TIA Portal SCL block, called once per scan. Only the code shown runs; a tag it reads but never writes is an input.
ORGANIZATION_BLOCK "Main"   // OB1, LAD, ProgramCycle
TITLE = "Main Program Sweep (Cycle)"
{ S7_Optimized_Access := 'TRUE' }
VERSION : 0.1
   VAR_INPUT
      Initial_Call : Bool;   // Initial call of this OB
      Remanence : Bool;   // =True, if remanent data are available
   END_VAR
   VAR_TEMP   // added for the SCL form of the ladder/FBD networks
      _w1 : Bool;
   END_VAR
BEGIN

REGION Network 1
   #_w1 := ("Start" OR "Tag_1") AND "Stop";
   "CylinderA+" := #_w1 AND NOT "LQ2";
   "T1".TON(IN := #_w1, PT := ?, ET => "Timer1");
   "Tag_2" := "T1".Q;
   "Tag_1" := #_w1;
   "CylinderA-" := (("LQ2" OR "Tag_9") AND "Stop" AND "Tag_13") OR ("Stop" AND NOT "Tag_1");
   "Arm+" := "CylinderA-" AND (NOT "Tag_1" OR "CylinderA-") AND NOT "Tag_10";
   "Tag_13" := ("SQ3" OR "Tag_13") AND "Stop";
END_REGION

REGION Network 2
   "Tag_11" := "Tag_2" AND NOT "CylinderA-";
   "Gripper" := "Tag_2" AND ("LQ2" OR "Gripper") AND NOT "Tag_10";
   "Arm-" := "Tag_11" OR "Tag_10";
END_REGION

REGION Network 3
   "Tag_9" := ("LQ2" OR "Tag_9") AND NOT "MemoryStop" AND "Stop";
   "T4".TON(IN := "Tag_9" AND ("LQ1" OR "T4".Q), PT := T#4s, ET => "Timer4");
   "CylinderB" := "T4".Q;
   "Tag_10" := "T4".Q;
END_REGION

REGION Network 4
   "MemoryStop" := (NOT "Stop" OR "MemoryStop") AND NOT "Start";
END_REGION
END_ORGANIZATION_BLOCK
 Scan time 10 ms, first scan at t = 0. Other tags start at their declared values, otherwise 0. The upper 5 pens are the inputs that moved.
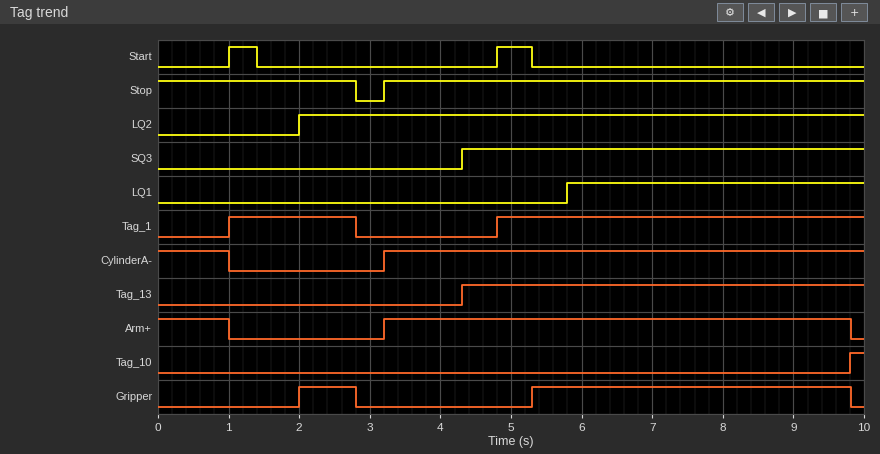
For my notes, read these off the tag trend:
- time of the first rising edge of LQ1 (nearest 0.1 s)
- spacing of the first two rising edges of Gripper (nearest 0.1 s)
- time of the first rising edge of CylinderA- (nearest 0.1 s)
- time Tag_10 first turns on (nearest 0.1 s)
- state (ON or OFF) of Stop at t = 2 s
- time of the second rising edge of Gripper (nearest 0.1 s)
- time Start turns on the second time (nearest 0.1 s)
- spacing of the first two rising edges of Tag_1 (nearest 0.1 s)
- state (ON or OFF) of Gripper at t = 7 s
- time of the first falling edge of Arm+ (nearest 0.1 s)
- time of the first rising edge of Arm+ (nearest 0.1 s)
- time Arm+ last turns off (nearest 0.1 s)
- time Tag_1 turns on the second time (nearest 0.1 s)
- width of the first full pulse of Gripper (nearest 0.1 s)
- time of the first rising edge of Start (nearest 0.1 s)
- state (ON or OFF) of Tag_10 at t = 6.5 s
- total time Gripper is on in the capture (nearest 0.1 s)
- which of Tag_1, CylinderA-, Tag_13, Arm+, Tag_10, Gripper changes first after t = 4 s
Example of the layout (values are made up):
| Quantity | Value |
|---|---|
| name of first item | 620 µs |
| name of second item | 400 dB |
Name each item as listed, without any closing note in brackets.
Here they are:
| Quantity | Value |
|---|---|
| time of the first rising edge of LQ1 | 5.8 s |
| spacing of the first two rising edges of Gripper | 3.3 s |
| time of the first rising edge of CylinderA- | 3.2 s |
| time Tag_10 first turns on | 9.8 s |
| state (ON or OFF) of Stop at t = 2 s | ON |
| time of the second rising edge of Gripper | 5.3 s |
| time Start turns on the second time | 4.8 s |
| spacing of the first two rising edges of Tag_1 | 3.8 s |
| state (ON or OFF) of Gripper at t = 7 s | ON |
| time of the first falling edge of Arm+ | 1.0 s |
| time of the first rising edge of Arm+ | 3.2 s |
| time Arm+ last turns off | 9.8 s |
| time Tag_1 turns on the second time | 4.8 s |
| width of the first full pulse of Gripper | 0.8 s |
| time of the first rising edge of Start | 1.0 s |
| state (ON or OFF) of Tag_10 at t = 6.5 s | OFF |
| total time Gripper is on in the capture | 5.3 s |
| which of Tag_1, CylinderA-, Tag_13, Arm+, Tag_10, Gripper changes first after t = 4 s | Tag_13 |
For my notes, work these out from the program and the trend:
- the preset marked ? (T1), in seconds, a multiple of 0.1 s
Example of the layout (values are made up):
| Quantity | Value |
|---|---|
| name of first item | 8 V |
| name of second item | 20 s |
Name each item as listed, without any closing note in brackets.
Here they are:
| Quantity | Value |
|---|---|
| the preset marked ? (T1), in seconds, a multiple of 0.1 s | 0.5 s |
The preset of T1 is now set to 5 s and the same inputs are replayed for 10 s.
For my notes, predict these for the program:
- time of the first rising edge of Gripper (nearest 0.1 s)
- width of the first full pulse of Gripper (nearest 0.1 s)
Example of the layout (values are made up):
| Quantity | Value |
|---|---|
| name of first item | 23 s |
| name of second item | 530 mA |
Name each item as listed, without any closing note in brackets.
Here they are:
| Quantity | Value |
|---|---|
| time of the first rising edge of Gripper | 9.8 s |
| width of the first full pulse of Gripper | 0.0 s |
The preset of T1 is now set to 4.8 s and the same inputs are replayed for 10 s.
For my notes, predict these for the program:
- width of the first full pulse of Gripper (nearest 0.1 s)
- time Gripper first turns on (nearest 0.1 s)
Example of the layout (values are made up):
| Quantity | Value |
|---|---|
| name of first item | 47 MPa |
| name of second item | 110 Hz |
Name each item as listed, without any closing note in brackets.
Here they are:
| Quantity | Value |
|---|---|
| width of the first full pulse of Gripper | 0.2 s |
| time Gripper first turns on | 9.6 s |
